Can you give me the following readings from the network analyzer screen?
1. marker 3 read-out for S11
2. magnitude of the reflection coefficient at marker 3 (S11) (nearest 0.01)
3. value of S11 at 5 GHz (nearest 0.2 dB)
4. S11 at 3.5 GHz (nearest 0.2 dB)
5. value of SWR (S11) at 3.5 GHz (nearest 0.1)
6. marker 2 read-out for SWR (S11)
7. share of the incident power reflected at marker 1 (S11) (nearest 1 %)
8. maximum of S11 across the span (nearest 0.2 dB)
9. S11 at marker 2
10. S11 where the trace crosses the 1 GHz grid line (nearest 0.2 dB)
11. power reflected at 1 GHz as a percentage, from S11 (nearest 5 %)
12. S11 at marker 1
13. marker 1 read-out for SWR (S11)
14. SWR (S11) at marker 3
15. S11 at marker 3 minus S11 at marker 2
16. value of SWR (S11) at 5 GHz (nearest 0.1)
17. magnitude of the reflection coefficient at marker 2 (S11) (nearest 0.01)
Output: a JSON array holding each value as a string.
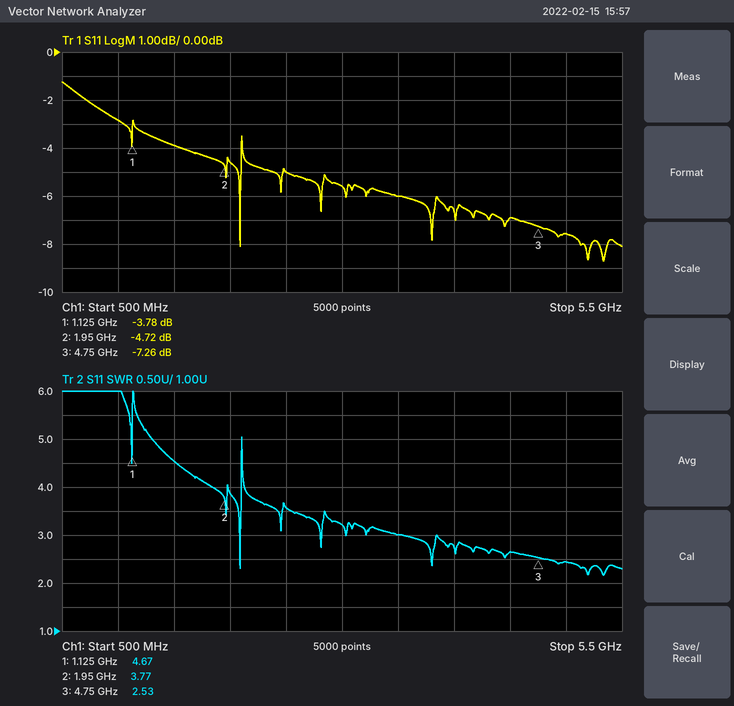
["-7.26 dB", "0.43", "-7.6 dB", "-6.0 dB", "3.0", "3.77", "42 %", "-1.2 dB", "-4.72 dB", "-2.8 dB", "50 %", "-3.78 dB", "4.67", "2.53", "-2.54 dB", "2.4", "0.58"]
